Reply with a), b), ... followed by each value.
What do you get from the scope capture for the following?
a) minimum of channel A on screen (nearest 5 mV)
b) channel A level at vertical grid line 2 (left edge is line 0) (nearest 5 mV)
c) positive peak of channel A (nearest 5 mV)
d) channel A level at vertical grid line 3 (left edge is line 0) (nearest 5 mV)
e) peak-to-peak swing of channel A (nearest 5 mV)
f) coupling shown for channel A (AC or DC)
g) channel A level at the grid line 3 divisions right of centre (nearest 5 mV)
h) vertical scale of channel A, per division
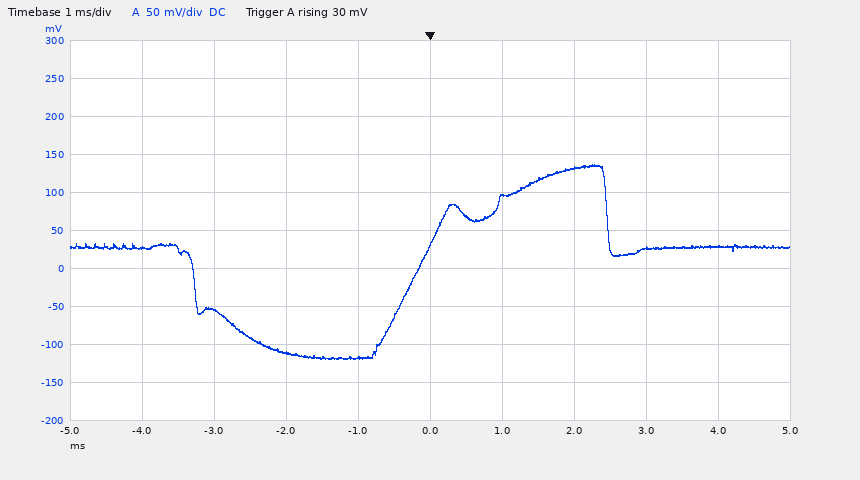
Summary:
a) -120 mV
b) -55 mV
c) 135 mV
d) -110 mV
e) 255 mV
f) DC
g) 25 mV
h) 50 mV
